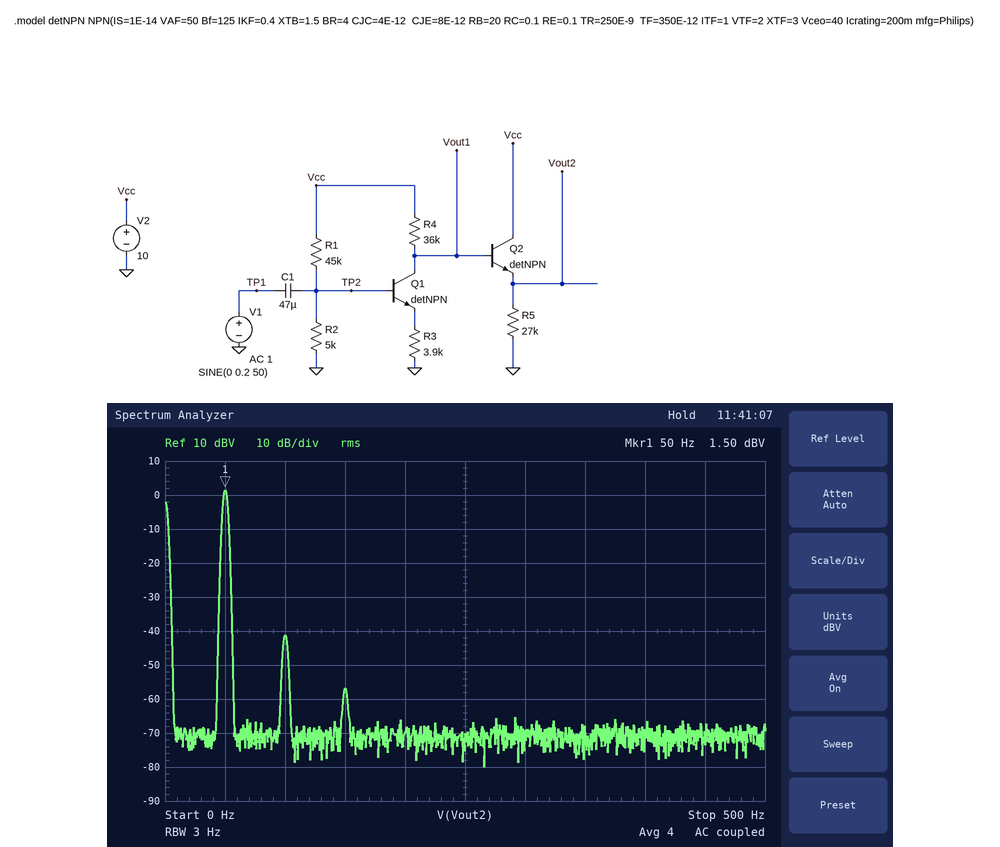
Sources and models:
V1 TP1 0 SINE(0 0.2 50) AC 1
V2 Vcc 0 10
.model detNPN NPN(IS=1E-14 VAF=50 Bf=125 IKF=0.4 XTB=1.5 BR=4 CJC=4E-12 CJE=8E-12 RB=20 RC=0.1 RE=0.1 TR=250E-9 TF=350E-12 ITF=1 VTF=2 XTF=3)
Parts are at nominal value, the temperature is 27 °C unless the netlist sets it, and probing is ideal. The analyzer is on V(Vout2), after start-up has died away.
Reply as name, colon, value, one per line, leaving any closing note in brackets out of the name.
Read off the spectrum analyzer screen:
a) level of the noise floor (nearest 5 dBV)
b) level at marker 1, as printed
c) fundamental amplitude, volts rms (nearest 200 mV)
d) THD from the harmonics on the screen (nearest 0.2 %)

level of the noise floor: -70 dBV
level at marker 1, as printed: 1.50 dBV
fundamental amplitude, volts rms: 1.2 V
THD from the harmonics on the screen: 0.8 %
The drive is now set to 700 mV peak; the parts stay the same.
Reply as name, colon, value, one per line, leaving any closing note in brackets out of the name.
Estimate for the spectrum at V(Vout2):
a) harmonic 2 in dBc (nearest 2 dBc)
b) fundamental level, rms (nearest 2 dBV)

harmonic 2 in dBc: -20 dBc
fundamental level, rms: 10 dBV
